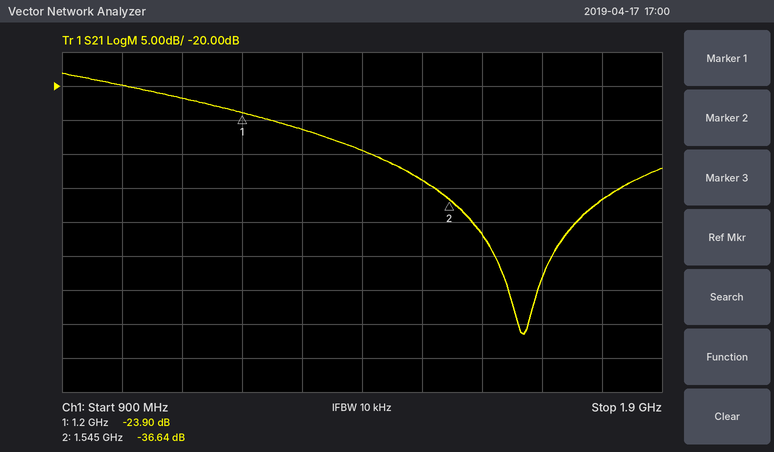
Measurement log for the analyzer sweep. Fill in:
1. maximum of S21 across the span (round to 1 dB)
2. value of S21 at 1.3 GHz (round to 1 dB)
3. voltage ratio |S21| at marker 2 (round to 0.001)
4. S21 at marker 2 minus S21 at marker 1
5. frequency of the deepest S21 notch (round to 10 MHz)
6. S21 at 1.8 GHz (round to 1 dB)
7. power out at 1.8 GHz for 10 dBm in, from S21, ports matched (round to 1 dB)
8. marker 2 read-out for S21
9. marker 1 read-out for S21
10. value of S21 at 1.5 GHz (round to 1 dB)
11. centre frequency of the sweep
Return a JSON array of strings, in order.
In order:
["-18 dB", "-26 dB", "0.015", "-12.74 dB", "1.67 GHz", "-37 dB", "-27 dBm", "-36.64 dB", "-23.90 dB", "-34 dB", "1.4 GHz"]
